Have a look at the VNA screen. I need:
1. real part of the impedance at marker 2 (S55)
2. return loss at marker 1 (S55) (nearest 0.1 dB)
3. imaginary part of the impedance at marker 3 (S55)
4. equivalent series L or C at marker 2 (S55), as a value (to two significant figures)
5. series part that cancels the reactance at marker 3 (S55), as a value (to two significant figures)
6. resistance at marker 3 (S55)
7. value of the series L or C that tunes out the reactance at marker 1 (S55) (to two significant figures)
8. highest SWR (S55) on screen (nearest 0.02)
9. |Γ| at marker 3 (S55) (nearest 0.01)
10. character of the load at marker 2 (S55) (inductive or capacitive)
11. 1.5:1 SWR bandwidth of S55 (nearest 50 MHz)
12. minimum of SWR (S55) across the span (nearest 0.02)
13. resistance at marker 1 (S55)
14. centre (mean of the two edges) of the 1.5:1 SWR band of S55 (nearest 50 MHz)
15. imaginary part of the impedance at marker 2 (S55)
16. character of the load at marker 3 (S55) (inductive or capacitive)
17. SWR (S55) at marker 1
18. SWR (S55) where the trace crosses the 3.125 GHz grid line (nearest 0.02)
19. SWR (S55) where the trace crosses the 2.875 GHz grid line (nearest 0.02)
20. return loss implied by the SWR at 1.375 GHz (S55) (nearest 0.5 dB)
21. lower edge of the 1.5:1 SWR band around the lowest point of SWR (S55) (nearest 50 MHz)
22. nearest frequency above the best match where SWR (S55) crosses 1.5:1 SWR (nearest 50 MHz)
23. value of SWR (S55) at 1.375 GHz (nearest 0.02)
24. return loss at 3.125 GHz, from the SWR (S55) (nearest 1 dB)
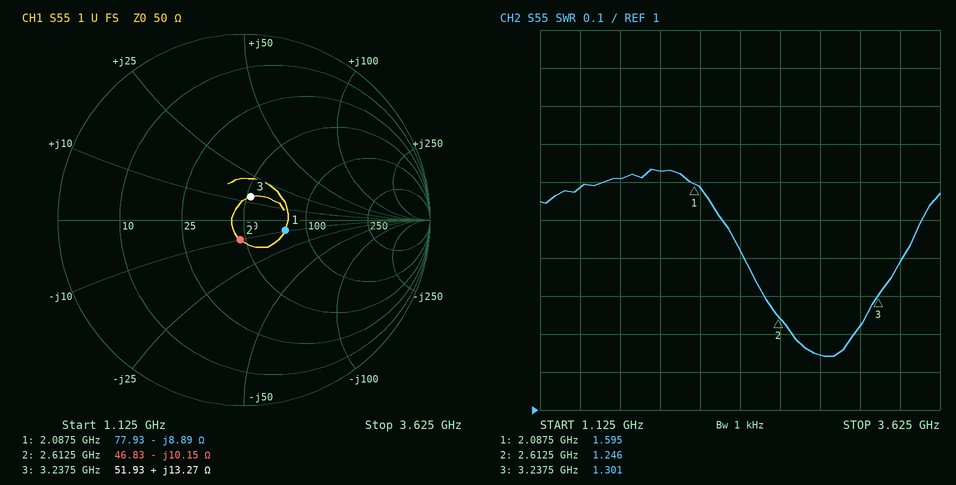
46.83 Ω
12.8 dB
+13.27 Ω
6.0 pF
3.7 pF
51.93 Ω
680 pH
1.64
0.13
capacitive
1.25 GHz
1.14
77.93 Ω
2.90 GHz
-10.15 Ω
inductive
1.595
1.22
1.14
13.0 dB
2.25 GHz
3.50 GHz
1.58
20 dB
